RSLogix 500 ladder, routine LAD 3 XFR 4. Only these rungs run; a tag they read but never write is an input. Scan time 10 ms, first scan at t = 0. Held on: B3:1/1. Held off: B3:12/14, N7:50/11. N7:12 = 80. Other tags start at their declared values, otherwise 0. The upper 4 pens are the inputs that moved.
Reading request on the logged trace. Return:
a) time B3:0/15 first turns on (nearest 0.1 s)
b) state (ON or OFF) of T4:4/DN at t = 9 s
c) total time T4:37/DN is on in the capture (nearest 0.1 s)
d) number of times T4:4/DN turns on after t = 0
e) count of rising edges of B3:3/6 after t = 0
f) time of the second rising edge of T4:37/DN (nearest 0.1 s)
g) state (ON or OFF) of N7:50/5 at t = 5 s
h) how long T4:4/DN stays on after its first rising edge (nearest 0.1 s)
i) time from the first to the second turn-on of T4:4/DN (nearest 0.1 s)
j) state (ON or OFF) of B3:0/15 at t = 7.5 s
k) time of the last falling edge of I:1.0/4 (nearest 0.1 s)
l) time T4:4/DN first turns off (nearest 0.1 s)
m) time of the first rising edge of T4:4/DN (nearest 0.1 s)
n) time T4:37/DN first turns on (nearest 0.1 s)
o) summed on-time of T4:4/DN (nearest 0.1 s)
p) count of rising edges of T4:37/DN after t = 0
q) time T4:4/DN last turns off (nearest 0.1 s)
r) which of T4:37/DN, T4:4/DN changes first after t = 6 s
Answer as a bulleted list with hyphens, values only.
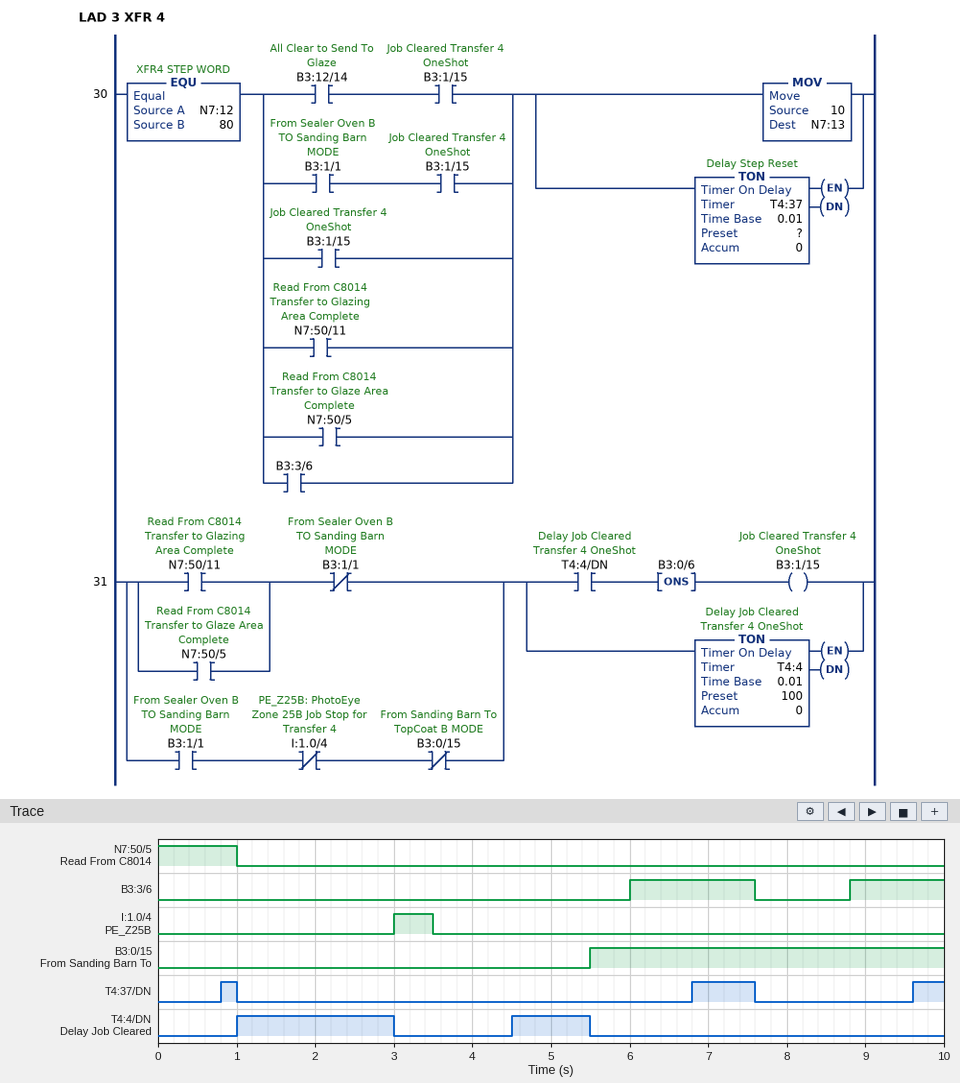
- 5.5 s
- OFF
- 1.4 s
- 2
- 2
- 6.8 s
- OFF
- 2.0 s
- 3.5 s
- ON
- 3.5 s
- 3.0 s
- 1.0 s
- 0.8 s
- 3.0 s
- 3
- 5.5 s
- T4:37/DN
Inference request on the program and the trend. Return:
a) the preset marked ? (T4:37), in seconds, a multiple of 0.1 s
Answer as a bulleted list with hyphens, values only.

- 0.8 s
